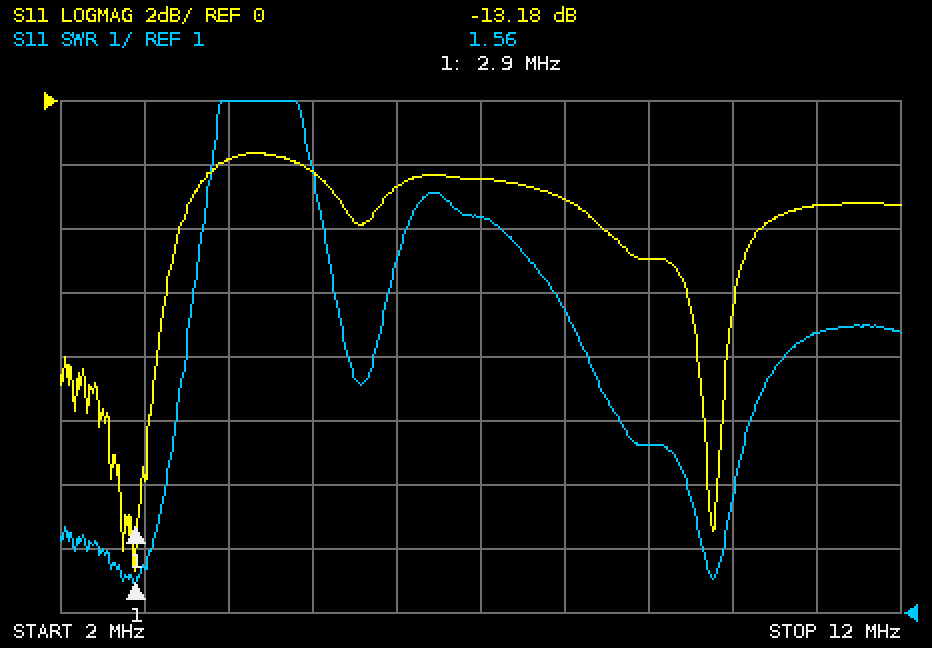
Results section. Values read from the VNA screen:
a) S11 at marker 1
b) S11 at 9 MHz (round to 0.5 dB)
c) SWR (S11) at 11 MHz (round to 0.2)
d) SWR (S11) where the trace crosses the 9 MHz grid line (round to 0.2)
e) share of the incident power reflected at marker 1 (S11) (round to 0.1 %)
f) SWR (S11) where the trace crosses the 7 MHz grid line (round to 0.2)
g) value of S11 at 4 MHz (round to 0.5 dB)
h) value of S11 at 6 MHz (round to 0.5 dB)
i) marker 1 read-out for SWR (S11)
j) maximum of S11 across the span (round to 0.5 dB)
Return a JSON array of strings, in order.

["-13.18 dB", "-5.0 dB", "5.4", "3.6", "4.8 %", "7.2", "-2.0 dB", "-2.5 dB", "1.56", "-1.5 dB"]
